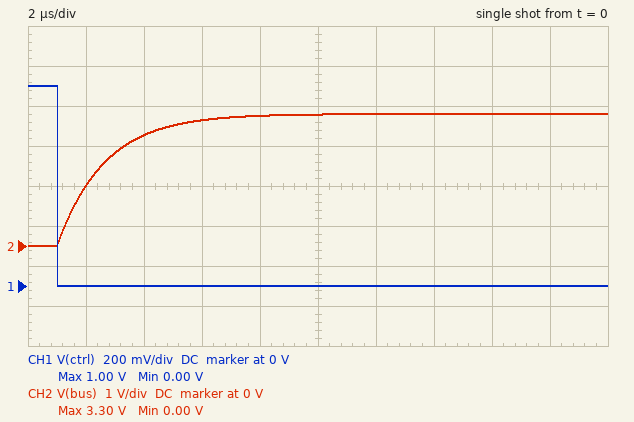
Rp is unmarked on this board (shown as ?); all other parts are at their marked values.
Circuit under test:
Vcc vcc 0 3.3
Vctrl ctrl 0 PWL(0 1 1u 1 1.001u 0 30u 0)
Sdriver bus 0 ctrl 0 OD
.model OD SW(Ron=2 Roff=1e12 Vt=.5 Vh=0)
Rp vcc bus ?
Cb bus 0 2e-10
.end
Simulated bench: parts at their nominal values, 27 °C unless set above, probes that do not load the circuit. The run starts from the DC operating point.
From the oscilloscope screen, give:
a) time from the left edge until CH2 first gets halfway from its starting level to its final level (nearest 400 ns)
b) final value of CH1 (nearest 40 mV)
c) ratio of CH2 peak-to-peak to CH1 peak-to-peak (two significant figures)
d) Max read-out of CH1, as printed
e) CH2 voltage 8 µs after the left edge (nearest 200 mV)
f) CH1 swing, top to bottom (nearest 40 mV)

2.0 µs
0 V
3.3
1.00 V
3.2 V
1.00 V
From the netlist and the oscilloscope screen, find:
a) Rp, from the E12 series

8.2 kΩ
